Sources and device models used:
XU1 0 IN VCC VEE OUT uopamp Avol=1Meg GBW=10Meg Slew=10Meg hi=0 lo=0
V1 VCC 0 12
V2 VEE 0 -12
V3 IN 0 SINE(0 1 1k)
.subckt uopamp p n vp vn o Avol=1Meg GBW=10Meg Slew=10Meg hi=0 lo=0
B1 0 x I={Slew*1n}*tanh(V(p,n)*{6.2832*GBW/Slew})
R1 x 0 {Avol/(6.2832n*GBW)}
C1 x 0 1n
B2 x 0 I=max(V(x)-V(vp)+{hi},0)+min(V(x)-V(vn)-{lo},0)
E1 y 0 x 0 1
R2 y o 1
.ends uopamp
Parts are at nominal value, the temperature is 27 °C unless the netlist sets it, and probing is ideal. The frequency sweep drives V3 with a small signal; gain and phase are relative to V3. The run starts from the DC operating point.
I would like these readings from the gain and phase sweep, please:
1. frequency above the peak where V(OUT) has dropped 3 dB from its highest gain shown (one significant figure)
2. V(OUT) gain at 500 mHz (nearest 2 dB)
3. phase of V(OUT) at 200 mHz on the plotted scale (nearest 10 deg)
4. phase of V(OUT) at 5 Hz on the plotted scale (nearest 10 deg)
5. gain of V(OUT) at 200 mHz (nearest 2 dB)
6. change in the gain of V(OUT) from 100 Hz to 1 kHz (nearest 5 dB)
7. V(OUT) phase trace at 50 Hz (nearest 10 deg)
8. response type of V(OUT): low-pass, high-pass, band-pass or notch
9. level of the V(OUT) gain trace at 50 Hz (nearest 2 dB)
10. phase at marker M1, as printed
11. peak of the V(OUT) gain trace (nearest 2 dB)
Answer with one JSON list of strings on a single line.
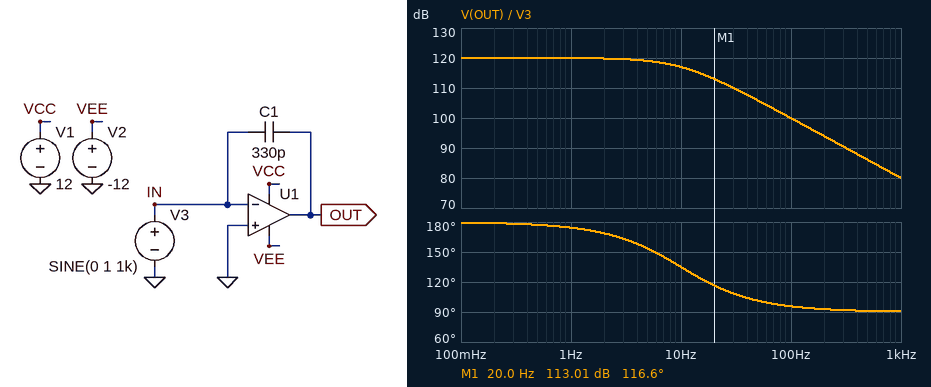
["10 Hz", "120 dB", "180 deg", "150 deg", "120 dB", "-20 dB", "100 deg", "low-pass", "106 dB", "116.6 deg", "120 dB"]
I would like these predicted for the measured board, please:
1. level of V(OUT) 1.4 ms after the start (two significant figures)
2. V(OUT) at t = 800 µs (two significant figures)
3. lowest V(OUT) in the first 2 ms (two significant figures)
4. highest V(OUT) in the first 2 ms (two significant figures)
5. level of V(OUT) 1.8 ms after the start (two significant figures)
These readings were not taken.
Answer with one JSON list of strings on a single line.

["-12 V", "12 V", "-12 V", "12 V", "12 V"]
